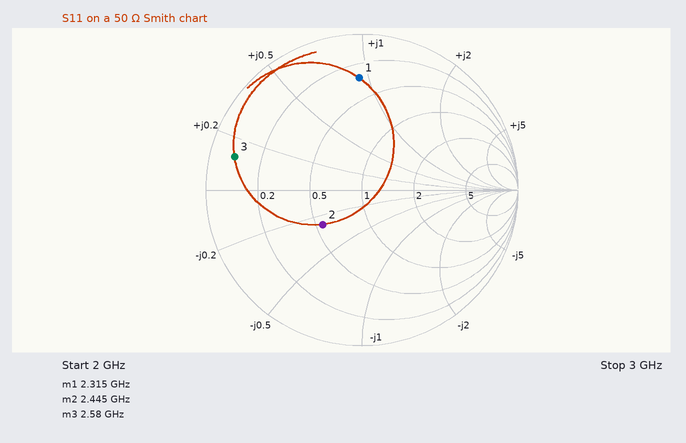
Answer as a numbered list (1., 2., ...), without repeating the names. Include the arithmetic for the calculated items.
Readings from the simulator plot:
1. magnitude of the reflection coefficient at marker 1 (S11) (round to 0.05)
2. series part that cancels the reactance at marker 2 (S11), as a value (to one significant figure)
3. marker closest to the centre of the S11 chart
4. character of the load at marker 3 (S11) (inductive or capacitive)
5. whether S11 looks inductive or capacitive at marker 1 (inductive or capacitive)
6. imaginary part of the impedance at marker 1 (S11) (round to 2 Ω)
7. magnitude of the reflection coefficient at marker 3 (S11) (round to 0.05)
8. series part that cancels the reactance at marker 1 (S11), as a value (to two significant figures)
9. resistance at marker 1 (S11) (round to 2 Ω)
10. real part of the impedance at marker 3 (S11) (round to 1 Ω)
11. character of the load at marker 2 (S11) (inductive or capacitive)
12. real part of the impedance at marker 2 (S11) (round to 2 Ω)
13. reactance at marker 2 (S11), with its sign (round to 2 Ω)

1. 0.70
2. L = 14 Ω/(2π × 2.445 GHz) ≈ 911 pH, so 900 pH to one significant figure
3. marker 2
4. inductive
5. inductive
6. +46 Ω
7. 0.85
8. C = 1/(2π × 2.315 GHz × 46 Ω) ≈ 1.5 pF
9. 16 Ω
10. 4 Ω
11. capacitive
12. 28 Ω
13. -14 Ω
